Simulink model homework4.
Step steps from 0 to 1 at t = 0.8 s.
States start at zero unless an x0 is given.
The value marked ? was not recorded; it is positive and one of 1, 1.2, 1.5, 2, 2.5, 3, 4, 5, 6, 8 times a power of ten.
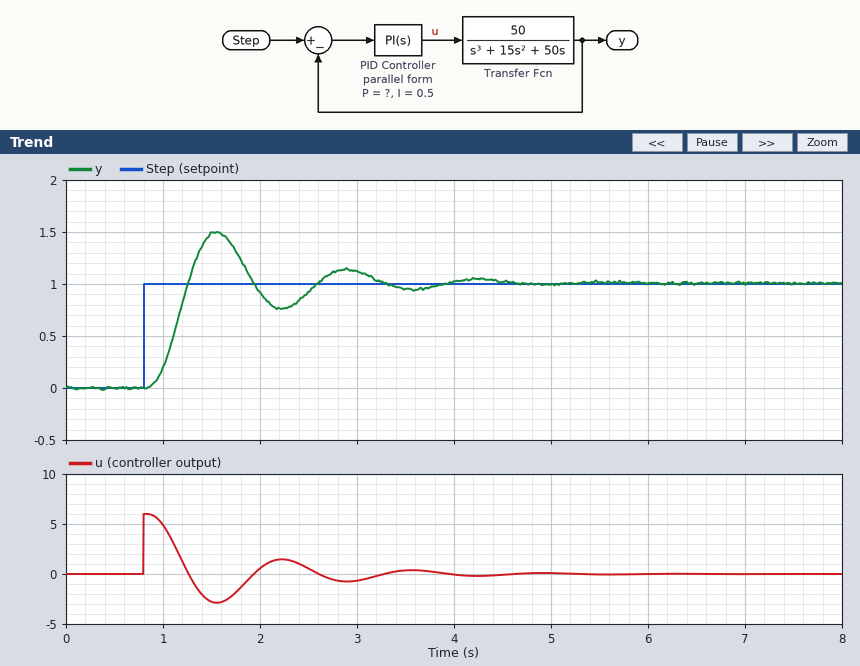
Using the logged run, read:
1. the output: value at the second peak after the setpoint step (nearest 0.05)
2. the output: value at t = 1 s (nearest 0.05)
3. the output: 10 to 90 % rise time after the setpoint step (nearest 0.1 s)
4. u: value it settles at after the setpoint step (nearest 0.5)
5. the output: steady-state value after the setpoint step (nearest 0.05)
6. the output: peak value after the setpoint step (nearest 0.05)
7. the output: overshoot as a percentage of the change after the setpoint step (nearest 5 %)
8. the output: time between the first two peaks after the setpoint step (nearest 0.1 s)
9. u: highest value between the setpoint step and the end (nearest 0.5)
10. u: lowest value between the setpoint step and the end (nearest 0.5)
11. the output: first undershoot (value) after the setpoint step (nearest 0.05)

1.15
0.20
0.3 s
0.0
1.00
1.50
50 %
1.3 s
6.0
-3.0
0.75
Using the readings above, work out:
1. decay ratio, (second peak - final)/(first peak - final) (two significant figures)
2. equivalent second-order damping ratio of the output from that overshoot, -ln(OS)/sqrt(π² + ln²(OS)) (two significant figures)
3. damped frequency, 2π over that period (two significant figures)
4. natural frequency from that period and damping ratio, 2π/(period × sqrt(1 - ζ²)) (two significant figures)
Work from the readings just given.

0.30
0.22
4.8 rad/s
5.0 rad/s
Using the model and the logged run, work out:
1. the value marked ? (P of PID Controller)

6
